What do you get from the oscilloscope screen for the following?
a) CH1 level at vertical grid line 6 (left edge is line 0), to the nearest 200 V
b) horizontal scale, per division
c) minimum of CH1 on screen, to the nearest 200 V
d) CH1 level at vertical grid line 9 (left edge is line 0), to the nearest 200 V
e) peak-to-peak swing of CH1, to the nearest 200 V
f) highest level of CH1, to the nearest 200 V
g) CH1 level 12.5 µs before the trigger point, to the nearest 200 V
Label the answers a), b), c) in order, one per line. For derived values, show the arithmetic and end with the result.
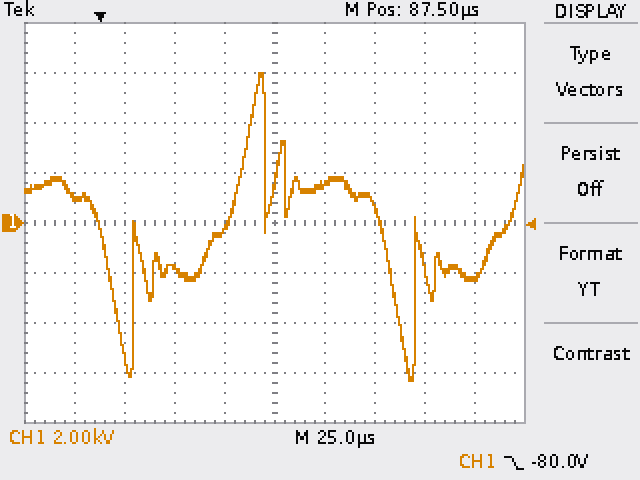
a) 1.6 kV
b) 25 µs
c) -6.4 kV
d) -2.2 kV
e) 6.0 kV − (-6.4 kV) = 12.4 kV
f) 6.0 kV
g) 1.0 kV
